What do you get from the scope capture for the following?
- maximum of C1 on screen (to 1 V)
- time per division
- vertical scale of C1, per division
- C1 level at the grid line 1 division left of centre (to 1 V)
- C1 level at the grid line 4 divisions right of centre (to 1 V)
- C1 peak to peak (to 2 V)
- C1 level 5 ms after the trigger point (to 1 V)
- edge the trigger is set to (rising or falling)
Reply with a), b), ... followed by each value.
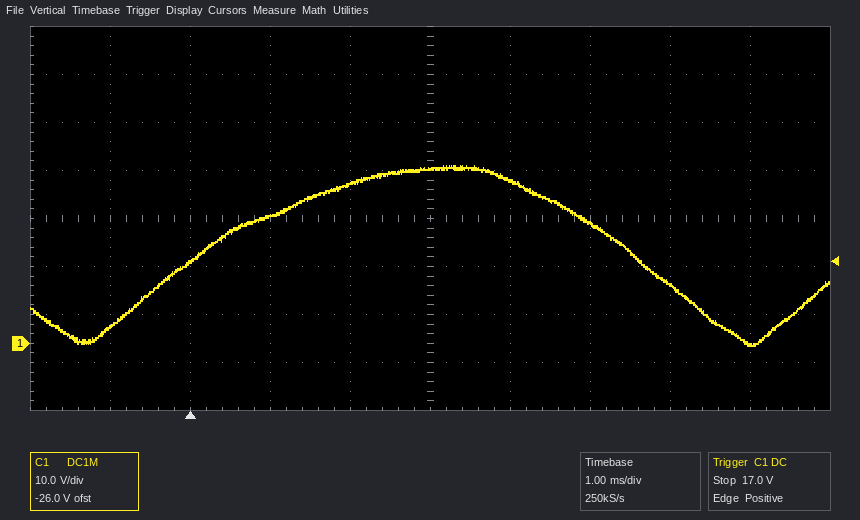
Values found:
a) 37 V
b) 1 ms
c) 10 V
d) 33 V
e) 0 V
f) 38 V
g) 25 V
h) rising
